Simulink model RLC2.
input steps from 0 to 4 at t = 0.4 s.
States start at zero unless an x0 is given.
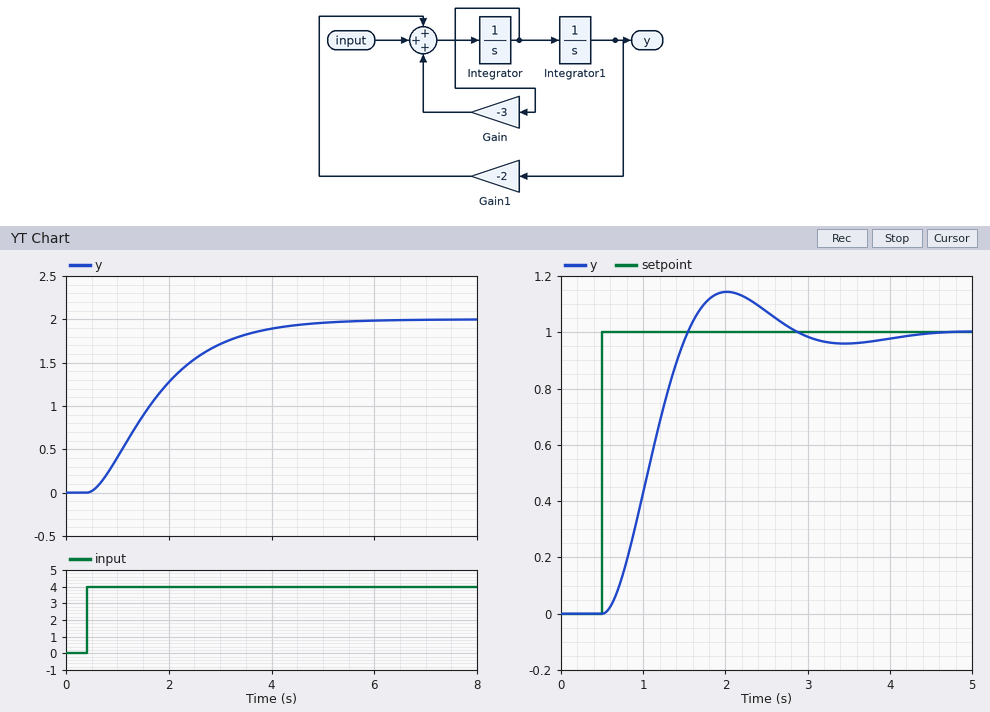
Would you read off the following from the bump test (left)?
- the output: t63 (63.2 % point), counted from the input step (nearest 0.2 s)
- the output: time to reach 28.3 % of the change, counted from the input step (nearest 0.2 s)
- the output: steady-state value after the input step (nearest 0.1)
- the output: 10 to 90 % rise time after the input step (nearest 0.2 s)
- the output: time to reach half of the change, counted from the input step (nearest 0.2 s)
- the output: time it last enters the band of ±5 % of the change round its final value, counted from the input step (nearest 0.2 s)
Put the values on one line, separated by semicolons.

1.6 s; 0.8 s; 2.0; 2.6 s; 1.2 s; 3.6 s
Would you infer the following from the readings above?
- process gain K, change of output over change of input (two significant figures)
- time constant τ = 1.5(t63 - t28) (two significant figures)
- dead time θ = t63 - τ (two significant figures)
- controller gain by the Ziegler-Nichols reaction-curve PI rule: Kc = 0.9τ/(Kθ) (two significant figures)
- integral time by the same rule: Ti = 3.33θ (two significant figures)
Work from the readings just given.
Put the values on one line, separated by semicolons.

0.50; 1.2 s; 0.40 s; 5.4; 1.3 s
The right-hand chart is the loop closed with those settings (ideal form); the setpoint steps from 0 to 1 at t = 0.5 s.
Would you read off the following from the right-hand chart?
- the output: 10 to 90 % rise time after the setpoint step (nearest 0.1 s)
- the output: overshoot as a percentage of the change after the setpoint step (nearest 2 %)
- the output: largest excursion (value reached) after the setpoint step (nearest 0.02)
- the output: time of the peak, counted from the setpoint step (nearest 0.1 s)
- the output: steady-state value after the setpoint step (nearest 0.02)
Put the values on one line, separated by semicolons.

0.7 s; 14 %; 1.14; 1.5 s; 1.00
